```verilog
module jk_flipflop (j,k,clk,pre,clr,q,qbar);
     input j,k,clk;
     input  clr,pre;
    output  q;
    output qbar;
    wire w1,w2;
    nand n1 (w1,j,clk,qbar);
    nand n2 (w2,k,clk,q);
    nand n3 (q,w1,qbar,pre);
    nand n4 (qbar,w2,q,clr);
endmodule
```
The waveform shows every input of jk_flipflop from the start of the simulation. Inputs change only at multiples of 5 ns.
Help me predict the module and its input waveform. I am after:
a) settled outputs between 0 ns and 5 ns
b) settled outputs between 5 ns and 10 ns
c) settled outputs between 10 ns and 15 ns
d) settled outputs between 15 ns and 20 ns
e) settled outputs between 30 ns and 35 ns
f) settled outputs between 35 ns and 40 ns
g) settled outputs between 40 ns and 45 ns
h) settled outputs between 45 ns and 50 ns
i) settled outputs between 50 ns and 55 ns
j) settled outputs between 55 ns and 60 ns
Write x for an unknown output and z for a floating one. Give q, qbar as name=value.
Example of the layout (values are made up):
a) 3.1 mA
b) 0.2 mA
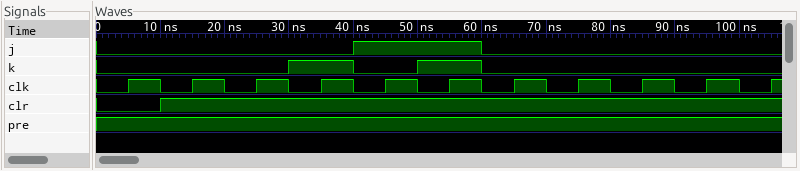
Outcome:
a) q=0, qbar=1
b) q=0, qbar=1
c) q=0, qbar=1
d) q=0, qbar=1
e) q=0, qbar=1
f) q=0, qbar=1
g) q=0, qbar=1
h) q=1, qbar=0
i) q=1, qbar=0
j) q=1, qbar=1
